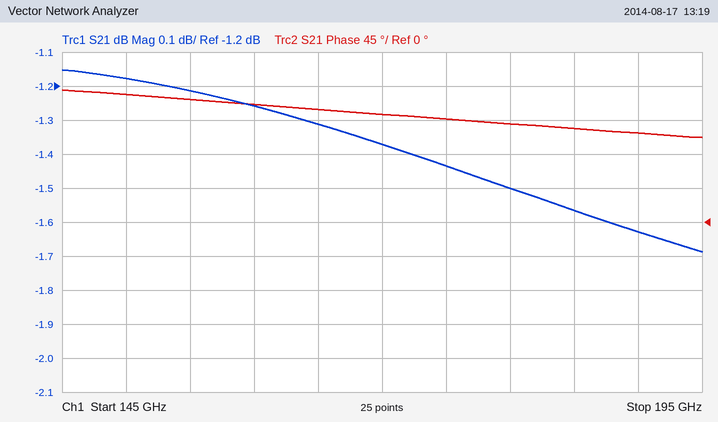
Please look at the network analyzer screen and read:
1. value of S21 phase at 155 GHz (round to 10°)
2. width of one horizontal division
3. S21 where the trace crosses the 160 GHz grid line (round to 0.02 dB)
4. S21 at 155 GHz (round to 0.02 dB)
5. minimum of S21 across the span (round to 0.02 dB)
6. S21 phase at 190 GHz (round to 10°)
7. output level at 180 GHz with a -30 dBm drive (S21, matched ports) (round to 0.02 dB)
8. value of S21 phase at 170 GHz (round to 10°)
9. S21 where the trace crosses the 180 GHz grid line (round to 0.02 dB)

160°
5 GHz
-1.26 dB
-1.22 dB
-1.68 dB
120°
-31.50 dBm
140°
-1.50 dB
